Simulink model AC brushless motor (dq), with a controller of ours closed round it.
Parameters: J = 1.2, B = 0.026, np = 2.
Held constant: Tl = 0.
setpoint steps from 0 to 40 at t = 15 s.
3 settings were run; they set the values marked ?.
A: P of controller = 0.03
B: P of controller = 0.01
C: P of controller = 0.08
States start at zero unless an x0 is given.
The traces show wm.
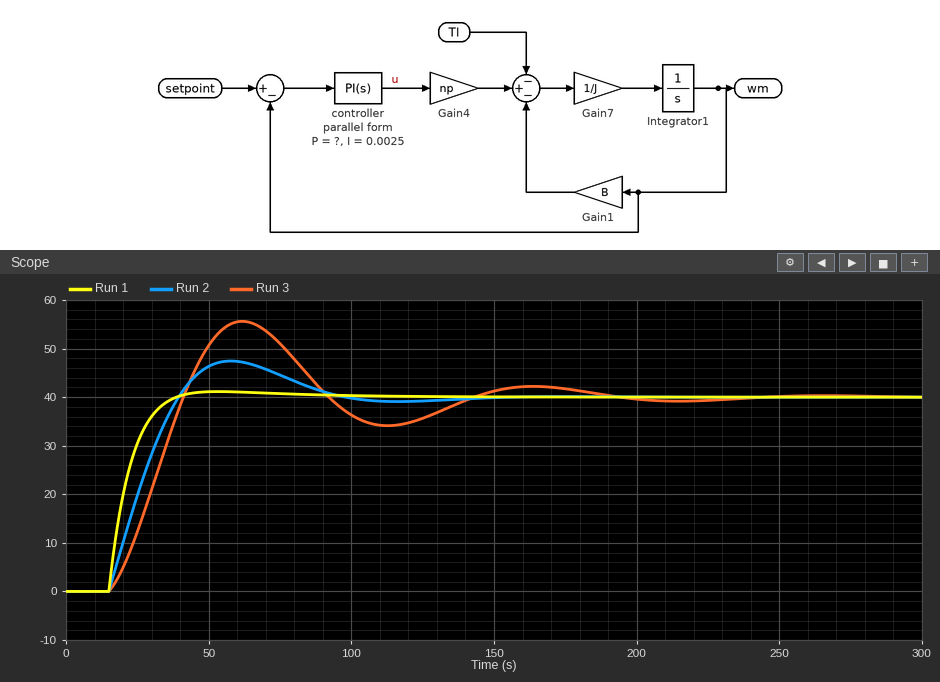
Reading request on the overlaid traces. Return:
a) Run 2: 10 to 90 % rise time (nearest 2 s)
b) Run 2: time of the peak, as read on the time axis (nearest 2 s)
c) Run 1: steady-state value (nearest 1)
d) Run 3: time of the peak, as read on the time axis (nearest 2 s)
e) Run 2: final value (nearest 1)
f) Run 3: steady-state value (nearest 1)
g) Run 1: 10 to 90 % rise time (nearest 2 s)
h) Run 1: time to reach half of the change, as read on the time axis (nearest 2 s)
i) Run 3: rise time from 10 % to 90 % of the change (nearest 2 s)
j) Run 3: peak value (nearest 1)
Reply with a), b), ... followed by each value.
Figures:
a) 18 s
b) 58 s
c) 40
d) 62 s
e) 40
f) 40
g) 14 s
h) 20 s
i) 20 s
j) 56
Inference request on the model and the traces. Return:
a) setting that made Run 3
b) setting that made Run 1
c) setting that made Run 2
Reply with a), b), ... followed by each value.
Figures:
a) B
b) C
c) A
